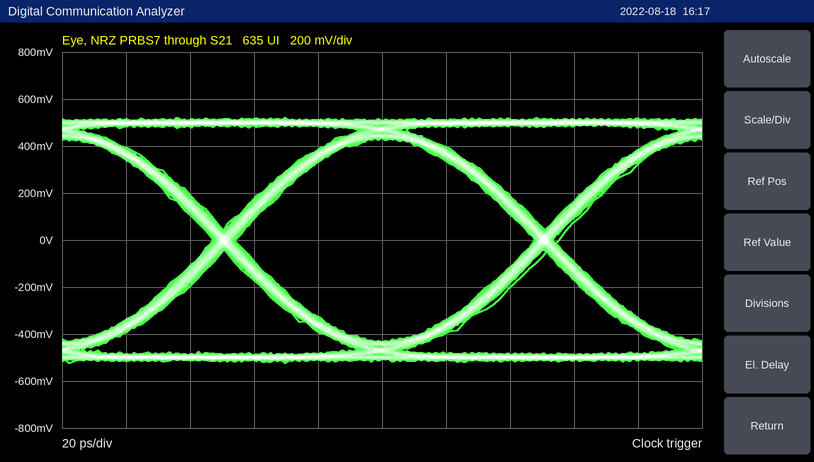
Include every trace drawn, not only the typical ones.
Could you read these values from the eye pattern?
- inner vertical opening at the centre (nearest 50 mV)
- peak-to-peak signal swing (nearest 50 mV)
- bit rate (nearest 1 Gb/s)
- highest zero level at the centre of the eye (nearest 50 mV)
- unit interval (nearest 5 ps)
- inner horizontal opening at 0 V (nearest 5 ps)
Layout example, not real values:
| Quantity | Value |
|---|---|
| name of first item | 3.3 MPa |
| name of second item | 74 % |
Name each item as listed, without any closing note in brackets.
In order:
| Quantity | Value |
|---|---|
| inner vertical opening at the centre | 850 mV |
| peak-to-peak signal swing | 1.05 V |
| bit rate | 10 Gb/s |
| highest zero level at the centre of the eye | -450 mV |
| unit interval | 100 ps |
| inner horizontal opening at 0 V | 95 ps |
